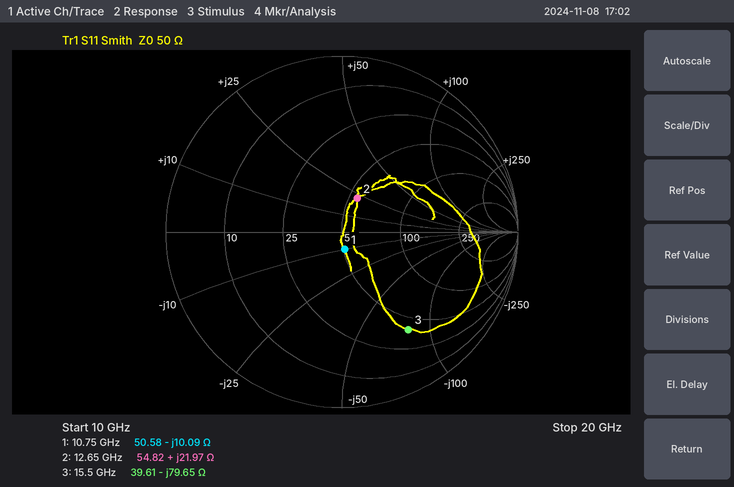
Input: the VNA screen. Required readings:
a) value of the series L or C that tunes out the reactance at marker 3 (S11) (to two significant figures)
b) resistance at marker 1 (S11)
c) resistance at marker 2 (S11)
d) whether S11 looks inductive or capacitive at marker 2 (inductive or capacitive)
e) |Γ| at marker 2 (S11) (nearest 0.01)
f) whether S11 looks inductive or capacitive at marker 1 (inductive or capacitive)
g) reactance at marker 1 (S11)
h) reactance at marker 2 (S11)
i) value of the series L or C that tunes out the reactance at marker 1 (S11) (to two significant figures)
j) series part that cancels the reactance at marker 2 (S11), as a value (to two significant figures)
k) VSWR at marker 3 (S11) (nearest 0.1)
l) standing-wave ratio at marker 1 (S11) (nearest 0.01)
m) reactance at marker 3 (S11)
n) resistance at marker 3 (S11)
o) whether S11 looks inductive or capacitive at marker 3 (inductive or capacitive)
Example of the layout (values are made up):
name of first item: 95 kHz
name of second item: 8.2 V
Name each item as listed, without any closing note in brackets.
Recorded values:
value of the series L or C that tunes out the reactance at marker 3 (S11): 820 pH
resistance at marker 1: 50.58 Ω
resistance at marker 2: 54.82 Ω
whether S11 looks inductive or capacitive at marker 2: inductive
|Γ| at marker 2 (S11): 0.21
whether S11 looks inductive or capacitive at marker 1: capacitive
reactance at marker 1: -10.09 Ω
reactance at marker 2: +21.97 Ω
value of the series L or C that tunes out the reactance at marker 1 (S11): 150 pH
series part that cancels the reactance at marker 2 (S11), as a value: 570 fF
VSWR at marker 3 (S11): 5.1
standing-wave ratio at marker 1 (S11): 1.22
reactance at marker 3: -79.65 Ω
resistance at marker 3: 39.61 Ω
whether S11 looks inductive or capacitive at marker 3: capacitive
